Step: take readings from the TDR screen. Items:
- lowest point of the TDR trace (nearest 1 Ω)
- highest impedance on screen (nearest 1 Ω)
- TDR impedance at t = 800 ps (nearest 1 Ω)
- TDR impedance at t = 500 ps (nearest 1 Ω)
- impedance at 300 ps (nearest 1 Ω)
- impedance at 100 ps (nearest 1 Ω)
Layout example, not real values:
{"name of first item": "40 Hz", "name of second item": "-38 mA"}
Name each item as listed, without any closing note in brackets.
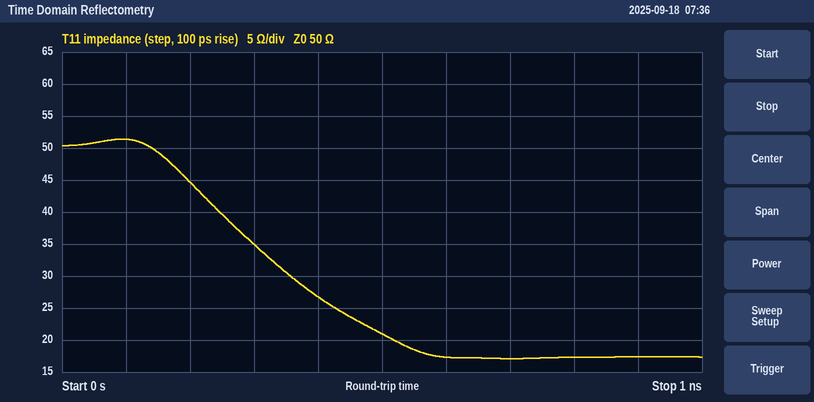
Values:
{"lowest point of the TDR trace": "17 Ω", "highest impedance on screen": "51 Ω", "TDR impedance at t = 800 ps": "17 Ω", "TDR impedance at t = 500 ps": "21 Ω", "impedance at 300 ps": "35 Ω", "impedance at 100 ps": "51 Ω"}
